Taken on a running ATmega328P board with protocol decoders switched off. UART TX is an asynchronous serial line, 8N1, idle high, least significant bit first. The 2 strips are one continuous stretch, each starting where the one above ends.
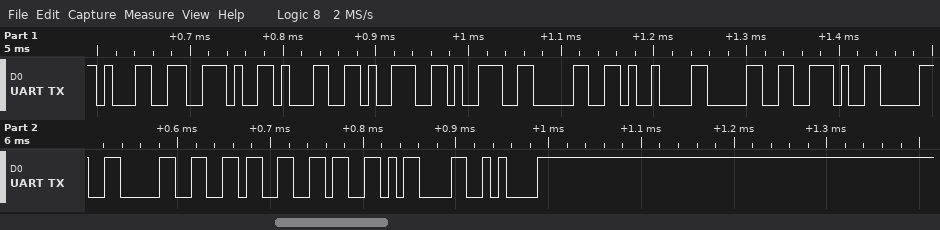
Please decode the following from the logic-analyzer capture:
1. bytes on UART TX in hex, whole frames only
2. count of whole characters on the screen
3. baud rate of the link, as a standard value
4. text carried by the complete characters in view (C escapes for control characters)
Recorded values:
31 2E 31 39 39 30 09 30 2E 30 30 36 36 0D 0A
15
115200 baud
"1.1990\t0.0066\r\n"
